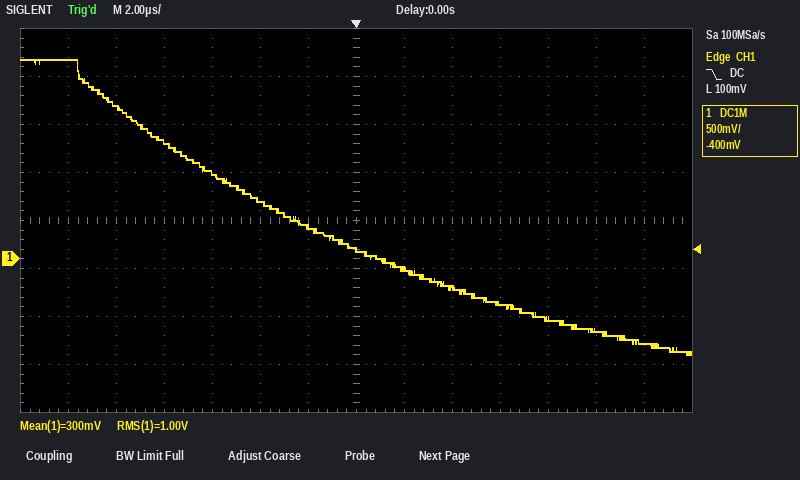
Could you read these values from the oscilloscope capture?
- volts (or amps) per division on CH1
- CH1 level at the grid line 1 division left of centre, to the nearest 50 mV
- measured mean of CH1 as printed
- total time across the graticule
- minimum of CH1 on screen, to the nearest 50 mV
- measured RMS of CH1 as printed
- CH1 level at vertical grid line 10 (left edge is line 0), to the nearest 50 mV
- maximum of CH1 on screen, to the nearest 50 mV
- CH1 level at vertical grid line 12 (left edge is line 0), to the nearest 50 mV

500 mV
350 mV
300 mV
28 µs
-1.00 V
1.00 V
-450 mV
2.10 V
-750 mV
